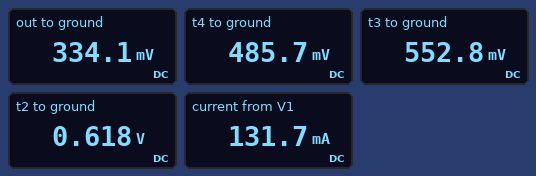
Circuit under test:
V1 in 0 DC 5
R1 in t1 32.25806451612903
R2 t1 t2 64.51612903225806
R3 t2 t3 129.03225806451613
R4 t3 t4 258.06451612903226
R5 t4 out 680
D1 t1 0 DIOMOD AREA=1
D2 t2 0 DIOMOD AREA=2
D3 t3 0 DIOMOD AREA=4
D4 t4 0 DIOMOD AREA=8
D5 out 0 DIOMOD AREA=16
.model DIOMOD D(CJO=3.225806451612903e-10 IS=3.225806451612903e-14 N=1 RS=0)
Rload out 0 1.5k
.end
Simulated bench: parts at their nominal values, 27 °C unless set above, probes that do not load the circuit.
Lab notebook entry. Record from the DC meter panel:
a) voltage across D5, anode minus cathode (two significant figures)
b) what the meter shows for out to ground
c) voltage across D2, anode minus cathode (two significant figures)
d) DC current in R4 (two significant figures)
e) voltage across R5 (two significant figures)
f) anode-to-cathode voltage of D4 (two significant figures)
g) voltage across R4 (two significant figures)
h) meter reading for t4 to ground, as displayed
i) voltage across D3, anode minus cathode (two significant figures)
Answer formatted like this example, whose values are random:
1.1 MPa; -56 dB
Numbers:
330 mV; 334.1 mV; 620 mV; 260 µA; 150 mV; 490 mV; 67 mV; 485.7 mV; 550 mV
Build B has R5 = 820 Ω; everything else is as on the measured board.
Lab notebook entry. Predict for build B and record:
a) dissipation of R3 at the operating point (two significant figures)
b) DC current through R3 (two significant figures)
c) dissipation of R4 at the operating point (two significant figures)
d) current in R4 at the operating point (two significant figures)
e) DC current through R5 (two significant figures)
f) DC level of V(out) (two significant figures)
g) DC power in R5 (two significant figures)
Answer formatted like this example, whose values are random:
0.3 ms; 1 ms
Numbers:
33 µW; 500 µA; 16 µW; 250 µA; 210 µA; 320 mV; 36 µW
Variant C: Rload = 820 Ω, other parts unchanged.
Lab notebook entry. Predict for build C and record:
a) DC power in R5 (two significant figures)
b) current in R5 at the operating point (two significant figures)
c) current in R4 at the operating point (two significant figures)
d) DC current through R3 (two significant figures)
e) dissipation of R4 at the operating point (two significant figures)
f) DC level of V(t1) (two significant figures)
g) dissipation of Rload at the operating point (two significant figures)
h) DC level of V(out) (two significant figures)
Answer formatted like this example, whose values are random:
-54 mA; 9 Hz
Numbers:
65 µW; 310 µA; 330 µA; 540 µA; 27 µW; 750 mV; 79 µW; 250 mV
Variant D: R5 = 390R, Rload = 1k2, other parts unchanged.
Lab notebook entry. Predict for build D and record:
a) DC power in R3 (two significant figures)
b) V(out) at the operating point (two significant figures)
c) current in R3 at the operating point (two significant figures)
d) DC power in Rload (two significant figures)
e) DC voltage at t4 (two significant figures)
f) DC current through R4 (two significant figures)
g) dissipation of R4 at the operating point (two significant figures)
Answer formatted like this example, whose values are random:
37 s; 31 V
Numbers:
36 µW; 350 mV; 530 µA; 100 µW; 470 mV; 310 µA; 25 µW
